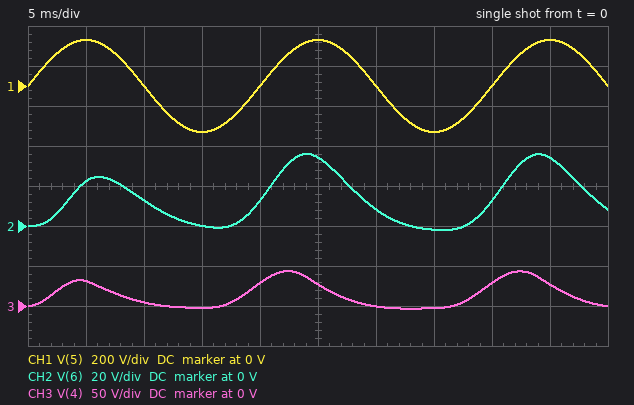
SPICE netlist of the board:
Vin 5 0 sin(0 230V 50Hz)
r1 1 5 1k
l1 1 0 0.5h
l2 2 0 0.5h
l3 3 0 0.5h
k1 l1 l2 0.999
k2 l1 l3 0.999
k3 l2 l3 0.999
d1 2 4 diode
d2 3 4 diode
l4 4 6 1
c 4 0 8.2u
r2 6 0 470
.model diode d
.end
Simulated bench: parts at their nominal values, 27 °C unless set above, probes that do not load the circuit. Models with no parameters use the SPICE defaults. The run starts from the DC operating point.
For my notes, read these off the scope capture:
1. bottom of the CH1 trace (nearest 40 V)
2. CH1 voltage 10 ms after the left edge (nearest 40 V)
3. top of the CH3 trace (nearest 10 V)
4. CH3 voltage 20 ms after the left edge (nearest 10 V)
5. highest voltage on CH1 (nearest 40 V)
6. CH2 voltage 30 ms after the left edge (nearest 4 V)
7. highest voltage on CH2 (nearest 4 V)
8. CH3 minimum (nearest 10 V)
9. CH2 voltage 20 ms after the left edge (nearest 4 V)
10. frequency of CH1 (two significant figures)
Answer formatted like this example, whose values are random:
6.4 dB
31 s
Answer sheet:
-240 V
0 V
40 V
30 V
240 V
8 V
36 V
0 V
12 V
50 Hz
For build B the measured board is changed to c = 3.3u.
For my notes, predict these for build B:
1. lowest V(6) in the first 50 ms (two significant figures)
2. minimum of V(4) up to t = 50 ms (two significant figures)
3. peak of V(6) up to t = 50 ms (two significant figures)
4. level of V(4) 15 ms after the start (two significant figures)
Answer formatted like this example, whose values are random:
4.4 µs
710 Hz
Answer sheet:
-5.4 V
-11 V
30 V
2.4 V
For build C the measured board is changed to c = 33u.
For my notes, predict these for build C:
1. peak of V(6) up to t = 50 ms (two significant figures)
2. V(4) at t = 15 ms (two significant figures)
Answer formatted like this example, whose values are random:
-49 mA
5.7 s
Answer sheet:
29 V
12 V
